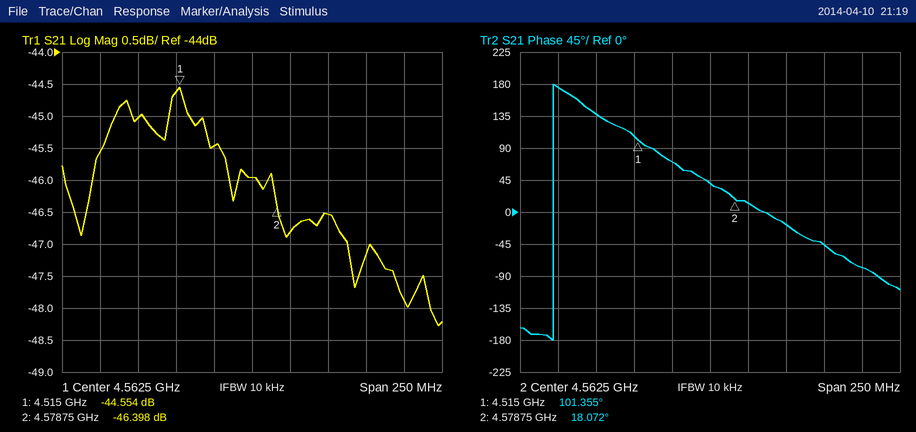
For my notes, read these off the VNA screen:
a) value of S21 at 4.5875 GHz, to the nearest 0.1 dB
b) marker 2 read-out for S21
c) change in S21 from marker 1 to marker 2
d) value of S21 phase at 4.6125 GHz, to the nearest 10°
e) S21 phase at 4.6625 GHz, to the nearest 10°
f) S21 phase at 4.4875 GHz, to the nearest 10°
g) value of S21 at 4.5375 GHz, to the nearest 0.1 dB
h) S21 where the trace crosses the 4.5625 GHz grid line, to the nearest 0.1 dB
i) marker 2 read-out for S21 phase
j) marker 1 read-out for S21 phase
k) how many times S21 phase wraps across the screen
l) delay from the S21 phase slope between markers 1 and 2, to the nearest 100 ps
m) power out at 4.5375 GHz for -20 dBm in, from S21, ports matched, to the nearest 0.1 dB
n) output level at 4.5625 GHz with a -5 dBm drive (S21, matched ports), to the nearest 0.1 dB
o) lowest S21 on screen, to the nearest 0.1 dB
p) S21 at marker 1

-46.8 dB
-46.398 dB
-1.844 dB
-20°
-80°
140°
-45.5 dB
-46.0 dB
18.072°
101.355°
1
3.6 ns
-65.5 dBm
-51.0 dBm
-48.3 dB
-44.554 dB
